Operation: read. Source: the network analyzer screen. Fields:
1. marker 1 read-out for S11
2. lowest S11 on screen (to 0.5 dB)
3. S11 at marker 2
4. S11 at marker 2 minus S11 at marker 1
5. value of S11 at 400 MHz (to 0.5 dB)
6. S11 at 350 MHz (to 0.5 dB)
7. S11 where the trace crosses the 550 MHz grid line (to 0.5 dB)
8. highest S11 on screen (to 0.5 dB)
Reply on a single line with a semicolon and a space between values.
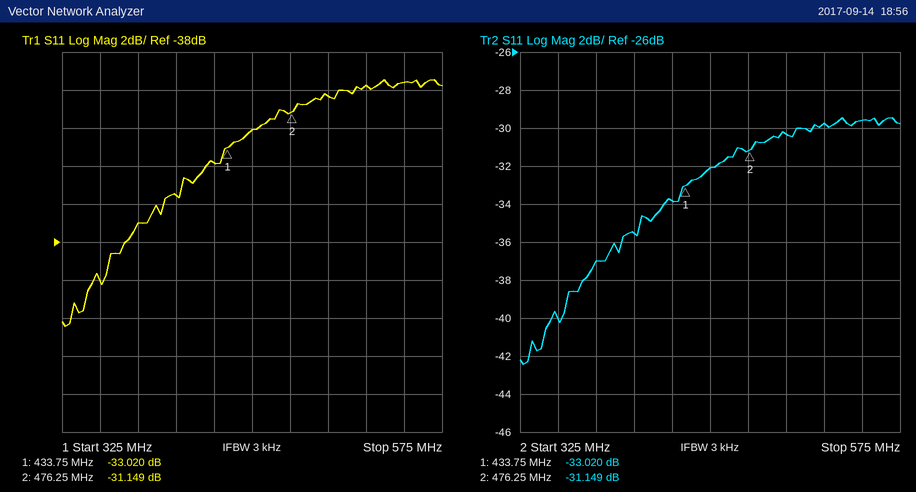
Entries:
-33.020 dB; -42.5 dB; -31.149 dB; 1.871 dB; -35.5 dB; -40.0 dB; -29.5 dB; -29.5 dB
